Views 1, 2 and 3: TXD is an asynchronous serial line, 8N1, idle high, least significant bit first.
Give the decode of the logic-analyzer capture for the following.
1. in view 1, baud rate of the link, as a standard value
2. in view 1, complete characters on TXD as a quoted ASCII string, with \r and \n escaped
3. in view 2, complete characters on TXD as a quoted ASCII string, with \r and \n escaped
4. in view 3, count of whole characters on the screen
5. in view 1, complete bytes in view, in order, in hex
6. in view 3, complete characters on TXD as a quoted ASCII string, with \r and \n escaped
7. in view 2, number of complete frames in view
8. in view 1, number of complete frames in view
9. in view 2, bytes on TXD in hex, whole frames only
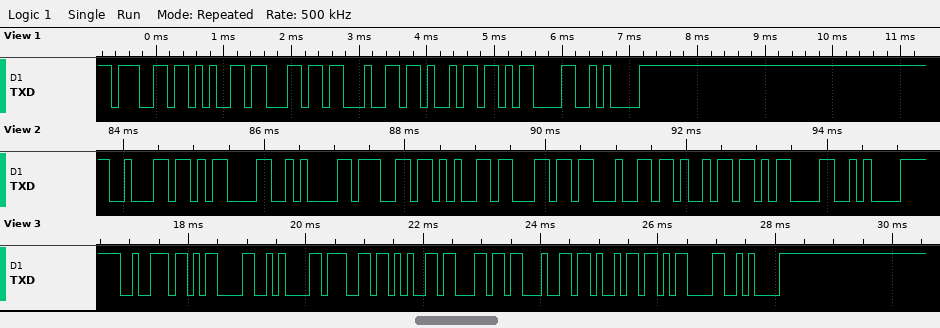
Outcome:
9600 baud
"geldi\r\n"
"b\r\ngeldi\r\n"
10
67 65 6C 64 69 0D 0A
"r\r\ngeldi\r\n"
10
7
62 0D 0A 67 65 6C 64 69 0D 0A
